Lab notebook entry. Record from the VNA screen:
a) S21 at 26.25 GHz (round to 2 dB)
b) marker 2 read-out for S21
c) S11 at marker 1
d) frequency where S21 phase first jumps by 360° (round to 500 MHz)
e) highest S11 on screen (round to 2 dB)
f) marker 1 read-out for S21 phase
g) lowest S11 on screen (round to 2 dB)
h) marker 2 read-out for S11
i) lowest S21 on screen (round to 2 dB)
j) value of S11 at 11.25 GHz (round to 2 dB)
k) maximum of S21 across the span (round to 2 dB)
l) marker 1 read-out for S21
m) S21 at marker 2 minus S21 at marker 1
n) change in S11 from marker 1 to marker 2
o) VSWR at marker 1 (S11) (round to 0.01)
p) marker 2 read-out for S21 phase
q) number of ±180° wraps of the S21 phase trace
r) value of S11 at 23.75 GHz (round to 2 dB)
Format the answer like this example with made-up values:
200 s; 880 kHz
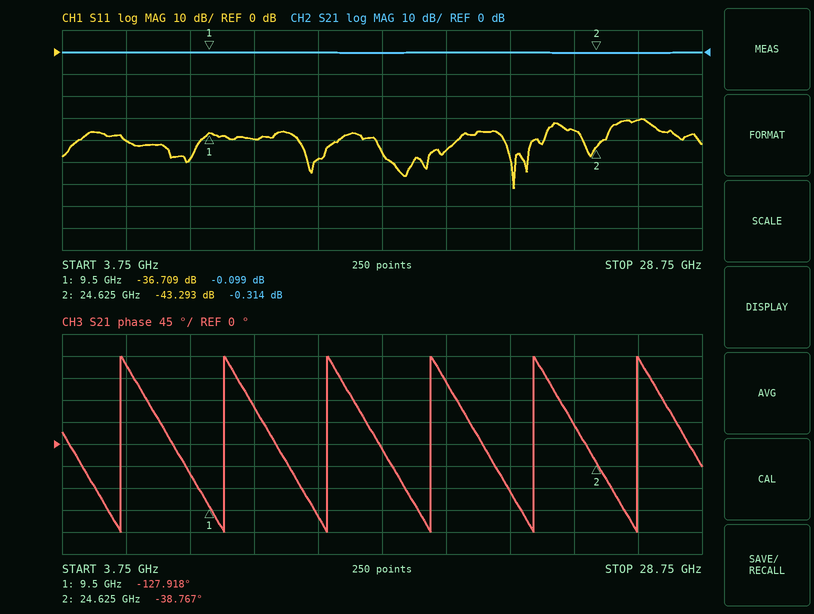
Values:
0 dB; -0.314 dB; -36.709 dB; 6.0 GHz; -30 dB; -127.918°; -62 dB; -43.293 dB; 0 dB; -40 dB; 0 dB; -0.099 dB; -0.215 dB; -6.584 dB; 1.03; -38.767°; 6; -36 dB
